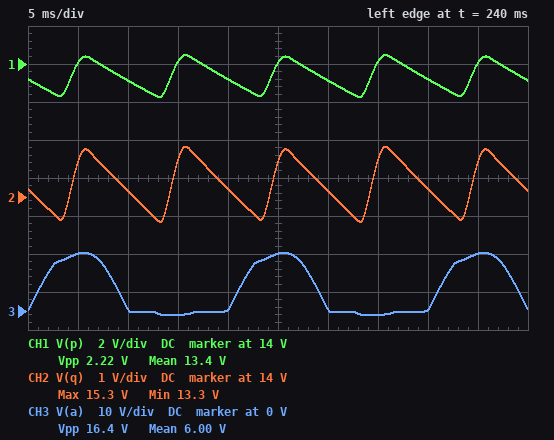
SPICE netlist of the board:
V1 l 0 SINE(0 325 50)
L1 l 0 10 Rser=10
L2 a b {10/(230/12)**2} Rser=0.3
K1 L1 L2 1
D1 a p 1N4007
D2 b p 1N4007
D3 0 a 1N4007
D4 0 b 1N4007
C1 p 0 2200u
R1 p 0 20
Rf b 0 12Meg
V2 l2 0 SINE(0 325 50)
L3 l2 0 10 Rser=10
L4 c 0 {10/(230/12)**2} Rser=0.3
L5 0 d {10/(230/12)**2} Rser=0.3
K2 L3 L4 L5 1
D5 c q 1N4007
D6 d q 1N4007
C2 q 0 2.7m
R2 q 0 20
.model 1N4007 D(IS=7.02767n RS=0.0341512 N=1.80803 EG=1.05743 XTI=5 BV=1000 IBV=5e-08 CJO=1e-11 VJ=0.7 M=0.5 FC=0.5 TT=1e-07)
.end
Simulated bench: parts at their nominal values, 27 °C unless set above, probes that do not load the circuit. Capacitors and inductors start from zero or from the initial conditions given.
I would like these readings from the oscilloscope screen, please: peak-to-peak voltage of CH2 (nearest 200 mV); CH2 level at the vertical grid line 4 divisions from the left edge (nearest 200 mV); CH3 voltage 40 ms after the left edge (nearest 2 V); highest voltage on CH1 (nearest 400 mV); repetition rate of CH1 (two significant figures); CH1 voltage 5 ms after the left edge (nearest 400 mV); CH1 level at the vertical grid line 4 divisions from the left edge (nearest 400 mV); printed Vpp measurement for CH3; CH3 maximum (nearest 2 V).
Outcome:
2.0 V
14.2 V
0 V
14.4 V
100 Hz
14.0 V
13.2 V
16.4 V
16 V
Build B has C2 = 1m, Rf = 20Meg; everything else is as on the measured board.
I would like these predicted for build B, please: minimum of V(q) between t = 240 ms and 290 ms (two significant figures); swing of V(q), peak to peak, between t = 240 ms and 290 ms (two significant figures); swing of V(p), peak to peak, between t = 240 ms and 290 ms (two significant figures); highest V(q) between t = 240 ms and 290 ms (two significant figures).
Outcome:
11 V
4.6 V
2.2 V
16 V
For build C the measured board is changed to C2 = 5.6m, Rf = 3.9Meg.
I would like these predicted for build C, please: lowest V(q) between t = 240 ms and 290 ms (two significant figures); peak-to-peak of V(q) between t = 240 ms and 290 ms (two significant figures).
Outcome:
14 V
990 mV
